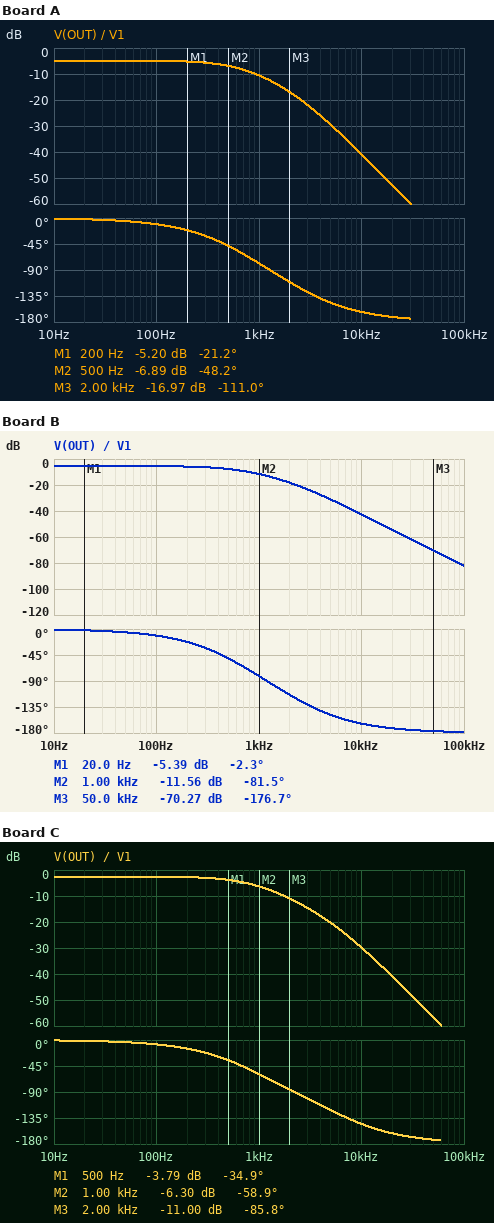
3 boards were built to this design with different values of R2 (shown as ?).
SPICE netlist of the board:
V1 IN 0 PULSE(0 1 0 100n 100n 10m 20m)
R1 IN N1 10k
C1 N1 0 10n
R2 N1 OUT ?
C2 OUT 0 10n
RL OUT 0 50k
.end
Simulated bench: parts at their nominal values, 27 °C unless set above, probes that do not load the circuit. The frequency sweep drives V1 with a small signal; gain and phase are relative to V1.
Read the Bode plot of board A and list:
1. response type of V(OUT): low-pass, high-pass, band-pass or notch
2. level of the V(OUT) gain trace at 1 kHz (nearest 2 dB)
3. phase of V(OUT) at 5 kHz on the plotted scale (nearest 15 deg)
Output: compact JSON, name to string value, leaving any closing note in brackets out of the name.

{"response type of V(OUT): low-pass, high-pass, band-pass or notch": "low-pass", "level of the V(OUT) gain trace at 1 kHz": "-10 dB", "phase of V(OUT) at 5 kHz on the plotted scale": "-150 deg"}
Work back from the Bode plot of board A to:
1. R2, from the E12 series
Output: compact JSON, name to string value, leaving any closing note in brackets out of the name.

{"R2, from the E12 series": "27 kΩ"}
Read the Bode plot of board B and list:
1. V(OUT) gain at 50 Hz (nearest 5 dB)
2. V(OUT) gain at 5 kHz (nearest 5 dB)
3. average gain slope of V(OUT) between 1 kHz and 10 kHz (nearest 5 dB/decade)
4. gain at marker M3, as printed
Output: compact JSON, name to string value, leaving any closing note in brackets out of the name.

{"V(OUT) gain at 50 Hz": "-5 dB", "V(OUT) gain at 5 kHz": "-30 dB", "average gain slope of V(OUT) between 1 kHz and 10 kHz": "-30 dB/decade", "gain at marker M3, as printed": "-70.27 dB"}
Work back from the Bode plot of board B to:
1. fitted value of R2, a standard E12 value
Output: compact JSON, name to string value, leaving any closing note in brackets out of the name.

{"fitted value of R2, a standard E12 value": "33 kΩ"}
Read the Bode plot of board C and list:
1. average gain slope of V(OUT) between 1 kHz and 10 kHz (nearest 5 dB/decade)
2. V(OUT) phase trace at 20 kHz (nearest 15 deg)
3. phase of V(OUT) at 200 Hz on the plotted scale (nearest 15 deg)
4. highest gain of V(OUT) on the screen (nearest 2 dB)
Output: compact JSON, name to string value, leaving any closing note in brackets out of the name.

{"average gain slope of V(OUT) between 1 kHz and 10 kHz": "-25 dB/decade", "V(OUT) phase trace at 20 kHz": "-165 deg", "phase of V(OUT) at 200 Hz on the plotted scale": "-15 deg", "highest gain of V(OUT) on the screen": "-2 dB"}
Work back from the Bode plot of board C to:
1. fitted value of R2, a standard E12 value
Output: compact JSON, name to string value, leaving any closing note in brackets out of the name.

{"fitted value of R2, a standard E12 value": "6.8 kΩ"}
